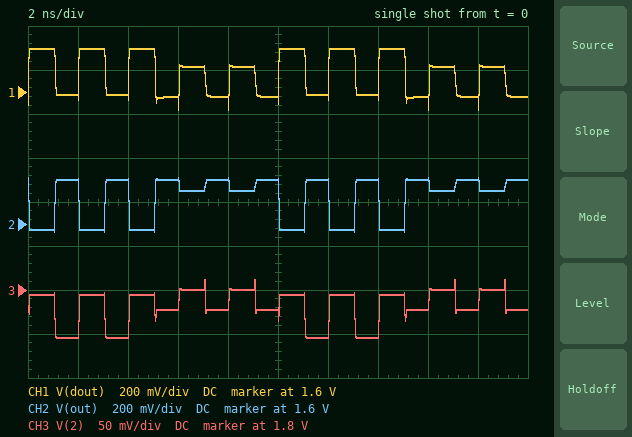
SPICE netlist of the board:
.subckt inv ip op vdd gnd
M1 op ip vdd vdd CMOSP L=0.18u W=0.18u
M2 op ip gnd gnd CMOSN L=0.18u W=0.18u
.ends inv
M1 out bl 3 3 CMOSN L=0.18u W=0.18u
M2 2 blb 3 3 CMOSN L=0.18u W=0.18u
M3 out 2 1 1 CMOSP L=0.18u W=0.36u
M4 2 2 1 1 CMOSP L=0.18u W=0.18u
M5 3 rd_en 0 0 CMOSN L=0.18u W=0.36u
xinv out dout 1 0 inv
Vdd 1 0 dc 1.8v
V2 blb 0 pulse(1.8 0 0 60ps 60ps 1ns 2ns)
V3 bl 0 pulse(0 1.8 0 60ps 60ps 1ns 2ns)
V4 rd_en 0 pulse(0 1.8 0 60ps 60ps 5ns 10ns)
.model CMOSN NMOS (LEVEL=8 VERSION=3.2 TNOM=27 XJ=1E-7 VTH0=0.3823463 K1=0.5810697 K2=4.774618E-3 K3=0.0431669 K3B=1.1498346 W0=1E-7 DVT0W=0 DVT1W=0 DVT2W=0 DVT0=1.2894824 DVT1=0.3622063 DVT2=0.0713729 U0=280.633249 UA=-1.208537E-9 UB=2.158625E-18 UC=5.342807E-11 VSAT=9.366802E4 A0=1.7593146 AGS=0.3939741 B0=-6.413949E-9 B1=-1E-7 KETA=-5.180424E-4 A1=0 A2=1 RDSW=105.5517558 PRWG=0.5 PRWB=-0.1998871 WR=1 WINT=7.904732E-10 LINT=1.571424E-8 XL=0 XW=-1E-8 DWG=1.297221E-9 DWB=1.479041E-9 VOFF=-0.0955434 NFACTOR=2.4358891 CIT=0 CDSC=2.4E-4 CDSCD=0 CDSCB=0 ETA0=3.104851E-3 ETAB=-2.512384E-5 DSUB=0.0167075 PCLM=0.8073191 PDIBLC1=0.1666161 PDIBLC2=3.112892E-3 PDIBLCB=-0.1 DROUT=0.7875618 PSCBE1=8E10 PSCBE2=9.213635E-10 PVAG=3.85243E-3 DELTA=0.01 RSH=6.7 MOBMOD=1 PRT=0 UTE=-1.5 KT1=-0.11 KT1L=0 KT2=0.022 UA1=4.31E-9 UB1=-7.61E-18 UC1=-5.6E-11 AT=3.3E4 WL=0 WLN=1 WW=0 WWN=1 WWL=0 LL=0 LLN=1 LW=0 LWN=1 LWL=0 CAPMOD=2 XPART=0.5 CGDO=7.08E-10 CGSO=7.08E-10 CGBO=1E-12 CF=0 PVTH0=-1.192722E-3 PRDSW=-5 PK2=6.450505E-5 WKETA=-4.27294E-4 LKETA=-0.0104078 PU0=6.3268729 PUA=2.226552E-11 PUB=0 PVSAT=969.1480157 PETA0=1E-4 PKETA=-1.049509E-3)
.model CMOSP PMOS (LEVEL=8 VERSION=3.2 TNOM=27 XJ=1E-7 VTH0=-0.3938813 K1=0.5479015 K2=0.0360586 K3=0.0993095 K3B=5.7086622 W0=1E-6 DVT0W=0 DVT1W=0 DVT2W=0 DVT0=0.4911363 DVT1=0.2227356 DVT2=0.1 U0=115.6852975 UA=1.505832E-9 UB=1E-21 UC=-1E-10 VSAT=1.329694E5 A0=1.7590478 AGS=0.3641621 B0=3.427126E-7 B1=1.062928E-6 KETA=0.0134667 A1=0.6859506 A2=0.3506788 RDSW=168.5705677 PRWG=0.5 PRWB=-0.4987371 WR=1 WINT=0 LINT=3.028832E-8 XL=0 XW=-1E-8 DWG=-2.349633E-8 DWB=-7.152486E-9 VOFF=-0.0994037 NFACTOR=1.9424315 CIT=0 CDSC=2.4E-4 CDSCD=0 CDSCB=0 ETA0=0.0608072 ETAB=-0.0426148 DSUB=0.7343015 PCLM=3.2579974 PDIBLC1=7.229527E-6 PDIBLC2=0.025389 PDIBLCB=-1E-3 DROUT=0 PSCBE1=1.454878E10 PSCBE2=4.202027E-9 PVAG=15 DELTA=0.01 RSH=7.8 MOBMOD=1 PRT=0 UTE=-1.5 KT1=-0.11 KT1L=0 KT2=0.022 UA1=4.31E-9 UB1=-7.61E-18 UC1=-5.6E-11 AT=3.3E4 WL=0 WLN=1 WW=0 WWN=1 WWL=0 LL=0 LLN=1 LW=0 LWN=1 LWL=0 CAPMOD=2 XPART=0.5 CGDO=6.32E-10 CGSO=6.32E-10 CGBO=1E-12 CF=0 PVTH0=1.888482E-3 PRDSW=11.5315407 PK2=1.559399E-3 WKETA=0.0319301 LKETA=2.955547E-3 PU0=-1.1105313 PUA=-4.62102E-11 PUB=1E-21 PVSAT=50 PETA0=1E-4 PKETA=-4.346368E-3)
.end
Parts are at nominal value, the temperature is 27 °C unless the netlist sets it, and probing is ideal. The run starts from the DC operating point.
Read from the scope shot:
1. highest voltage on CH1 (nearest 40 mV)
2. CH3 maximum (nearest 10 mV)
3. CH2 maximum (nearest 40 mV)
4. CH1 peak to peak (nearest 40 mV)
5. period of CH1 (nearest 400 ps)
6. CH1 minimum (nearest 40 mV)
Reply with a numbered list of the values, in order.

1. 1.80 V
2. 1.81 V
3. 1.80 V
4. 280 mV
5. 2.0 ns
6. 1.52 V
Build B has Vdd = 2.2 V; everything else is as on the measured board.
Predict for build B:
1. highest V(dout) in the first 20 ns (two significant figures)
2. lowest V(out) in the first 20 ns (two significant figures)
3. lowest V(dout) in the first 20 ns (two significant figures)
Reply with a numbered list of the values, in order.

1. 2.2 V
2. 2.0 V
3. 1.9 V
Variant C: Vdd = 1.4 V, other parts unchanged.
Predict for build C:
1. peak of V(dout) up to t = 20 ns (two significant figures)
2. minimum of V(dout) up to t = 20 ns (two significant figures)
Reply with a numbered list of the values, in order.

1. 1.4 V
2. 1.2 V
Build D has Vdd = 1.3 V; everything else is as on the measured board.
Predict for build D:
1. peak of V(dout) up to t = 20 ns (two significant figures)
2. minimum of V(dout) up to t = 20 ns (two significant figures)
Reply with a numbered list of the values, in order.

1. 1.3 V
2. 1.1 V
